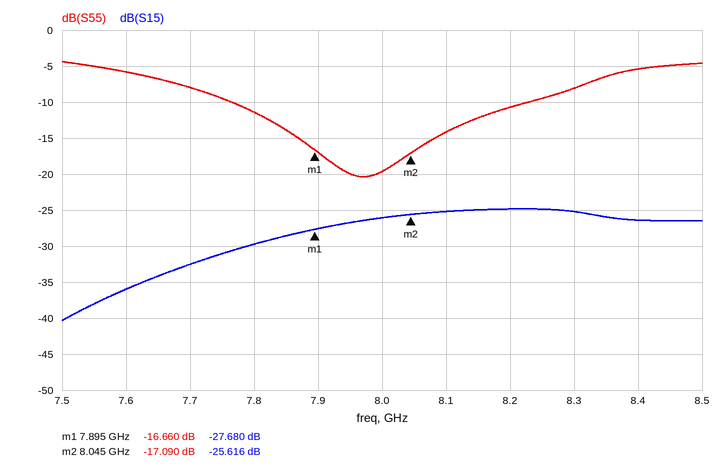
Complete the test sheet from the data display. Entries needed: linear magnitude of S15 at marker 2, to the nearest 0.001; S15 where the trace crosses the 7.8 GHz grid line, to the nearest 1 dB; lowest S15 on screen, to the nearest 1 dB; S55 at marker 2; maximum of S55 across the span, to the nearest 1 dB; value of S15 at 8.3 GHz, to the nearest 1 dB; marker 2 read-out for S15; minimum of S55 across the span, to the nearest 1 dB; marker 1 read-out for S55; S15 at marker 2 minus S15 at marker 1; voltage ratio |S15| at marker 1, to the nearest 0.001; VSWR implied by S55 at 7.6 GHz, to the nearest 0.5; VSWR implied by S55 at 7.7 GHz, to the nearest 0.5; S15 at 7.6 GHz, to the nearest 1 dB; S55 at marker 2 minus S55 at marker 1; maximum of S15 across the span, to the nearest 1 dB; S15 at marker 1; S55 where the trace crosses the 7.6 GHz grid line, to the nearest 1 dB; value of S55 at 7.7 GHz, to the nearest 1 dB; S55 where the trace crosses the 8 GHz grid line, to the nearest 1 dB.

0.052
-30 dB
-40 dB
-17.090 dB
-4 dB
-25 dB
-25.616 dB
-20 dB
-16.660 dB
2.064 dB
0.041
3.0
2.5
-36 dB
-0.430 dB
-25 dB
-27.680 dB
-6 dB
-8 dB
-20 dB
